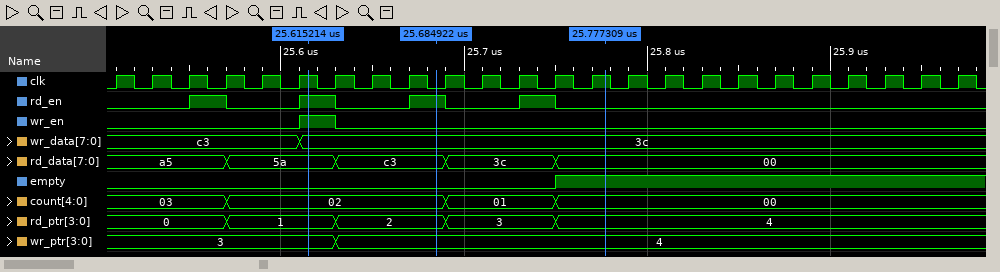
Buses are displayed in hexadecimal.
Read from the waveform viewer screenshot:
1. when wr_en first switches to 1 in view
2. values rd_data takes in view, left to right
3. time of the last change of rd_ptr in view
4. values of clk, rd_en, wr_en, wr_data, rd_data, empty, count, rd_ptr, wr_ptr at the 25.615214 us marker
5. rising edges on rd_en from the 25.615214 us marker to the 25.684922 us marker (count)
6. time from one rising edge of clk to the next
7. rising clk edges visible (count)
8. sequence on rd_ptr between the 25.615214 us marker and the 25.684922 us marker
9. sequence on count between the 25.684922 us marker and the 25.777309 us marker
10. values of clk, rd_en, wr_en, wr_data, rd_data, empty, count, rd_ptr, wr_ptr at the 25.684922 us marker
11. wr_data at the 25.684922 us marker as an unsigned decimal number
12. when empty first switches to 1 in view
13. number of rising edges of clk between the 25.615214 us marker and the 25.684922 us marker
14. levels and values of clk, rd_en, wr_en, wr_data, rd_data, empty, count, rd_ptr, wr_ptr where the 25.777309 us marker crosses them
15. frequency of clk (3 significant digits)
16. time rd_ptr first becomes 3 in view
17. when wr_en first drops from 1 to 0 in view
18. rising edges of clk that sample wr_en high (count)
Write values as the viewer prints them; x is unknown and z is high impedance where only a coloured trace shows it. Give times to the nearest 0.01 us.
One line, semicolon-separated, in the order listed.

25.61 us; a5, 5a, c3, 3c, 00; 25.75 us; clk=1, rd_en=1, wr_en=1, wr_data=3c, rd_data=5a, empty=0, count=02, rd_ptr=1, wr_ptr=3; 1; 0.02 us; 24; 1, 2; 02, 01, 00; clk=0, rd_en=1, wr_en=0, wr_data=3c, rd_data=c3, empty=0, count=02, rd_ptr=2, wr_ptr=4; 60; 25.75 us; 3; clk=1, rd_en=0, wr_en=0, wr_data=3c, rd_data=00, empty=1, count=00, rd_ptr=4, wr_ptr=4; 50.0 MHz; 25.69 us; 25.63 us; 1
